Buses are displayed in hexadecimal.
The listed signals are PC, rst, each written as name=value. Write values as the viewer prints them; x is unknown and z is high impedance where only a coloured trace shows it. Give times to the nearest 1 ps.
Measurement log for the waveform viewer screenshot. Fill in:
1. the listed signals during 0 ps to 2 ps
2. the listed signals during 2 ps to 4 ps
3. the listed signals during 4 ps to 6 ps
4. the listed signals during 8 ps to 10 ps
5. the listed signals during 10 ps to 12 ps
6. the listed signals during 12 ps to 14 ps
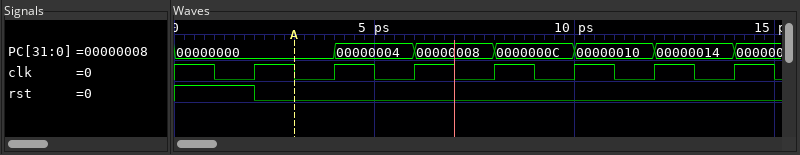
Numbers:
PC=00000000, rst=1
PC=00000000, rst=0
PC=00000004, rst=0
PC=0000000C, rst=0
PC=00000010, rst=0
PC=00000014, rst=0
